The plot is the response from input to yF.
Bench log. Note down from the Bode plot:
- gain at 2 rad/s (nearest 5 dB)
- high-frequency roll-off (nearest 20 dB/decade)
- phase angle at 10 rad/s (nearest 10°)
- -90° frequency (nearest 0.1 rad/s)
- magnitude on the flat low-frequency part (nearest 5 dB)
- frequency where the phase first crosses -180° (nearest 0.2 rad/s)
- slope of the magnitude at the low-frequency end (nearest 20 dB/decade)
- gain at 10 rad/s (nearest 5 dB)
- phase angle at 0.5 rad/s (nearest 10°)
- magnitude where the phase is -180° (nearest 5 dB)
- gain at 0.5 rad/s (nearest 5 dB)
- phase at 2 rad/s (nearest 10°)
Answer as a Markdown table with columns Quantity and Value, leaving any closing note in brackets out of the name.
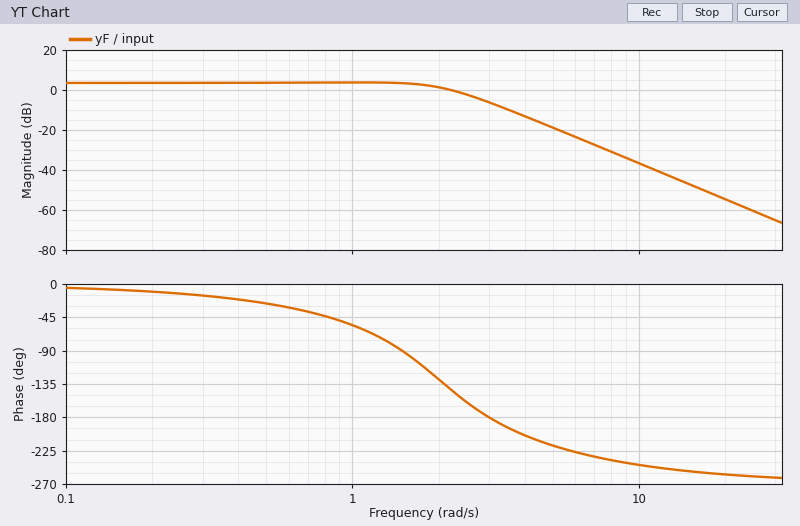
| Quantity | Value |
|---|---|
| gain at 2 rad/s | 0 dB |
| high-frequency roll-off | -60 dB/decade |
| phase angle at 10 rad/s | -240° |
| -90° frequency | 1.5 rad/s |
| magnitude on the flat low-frequency part | 5 dB |
| frequency where the phase first crosses -180° | 3.0 rad/s |
| slope of the magnitude at the low-frequency end | 0 dB/decade |
| gain at 10 rad/s | -35 dB |
| phase angle at 0.5 rad/s | -30° |
| magnitude where the phase is -180° | -5 dB |
| gain at 0.5 rad/s | 5 dB |
| phase at 2 rad/s | -130° |
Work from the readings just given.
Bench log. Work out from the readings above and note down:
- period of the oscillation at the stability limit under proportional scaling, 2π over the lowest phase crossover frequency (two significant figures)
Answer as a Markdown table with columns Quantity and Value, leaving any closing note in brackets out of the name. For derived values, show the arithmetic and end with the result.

| Quantity | Value |
|---|---|
| period of the oscillation at the stability limit under proportional scaling, 2π over the lowest phase crossover frequency | 2π / 3 = 2.1 s |
